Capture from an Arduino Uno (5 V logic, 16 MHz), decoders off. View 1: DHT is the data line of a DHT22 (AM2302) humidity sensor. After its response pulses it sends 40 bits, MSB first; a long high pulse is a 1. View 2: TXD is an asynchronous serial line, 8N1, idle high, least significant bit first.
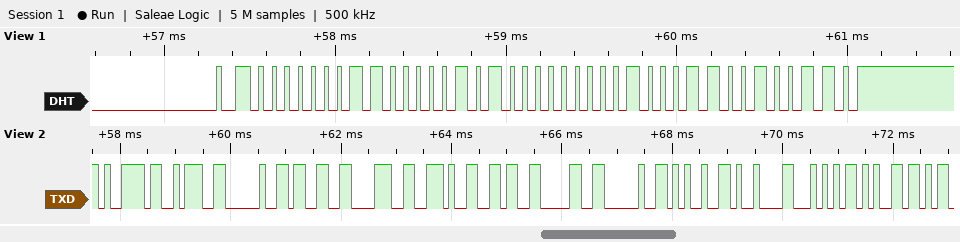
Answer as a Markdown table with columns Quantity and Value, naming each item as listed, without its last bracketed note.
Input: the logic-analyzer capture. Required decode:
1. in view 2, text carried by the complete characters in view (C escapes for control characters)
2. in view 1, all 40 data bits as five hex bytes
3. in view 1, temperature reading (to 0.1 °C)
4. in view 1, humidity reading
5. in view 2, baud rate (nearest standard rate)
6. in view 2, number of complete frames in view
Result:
| Quantity | Value |
|---|---|
| in view 2, text carried by the complete characters in view | "y: 38.60 %\tTe" |
| in view 1, all 40 data bits as five hex bytes | 01 82 80 23 26 |
| in view 1, temperature reading | -3.5 °C |
| in view 1, humidity reading | 38.6 % |
| in view 2, baud rate | 9600 baud |
| in view 2, number of complete frames in view | 13 |
